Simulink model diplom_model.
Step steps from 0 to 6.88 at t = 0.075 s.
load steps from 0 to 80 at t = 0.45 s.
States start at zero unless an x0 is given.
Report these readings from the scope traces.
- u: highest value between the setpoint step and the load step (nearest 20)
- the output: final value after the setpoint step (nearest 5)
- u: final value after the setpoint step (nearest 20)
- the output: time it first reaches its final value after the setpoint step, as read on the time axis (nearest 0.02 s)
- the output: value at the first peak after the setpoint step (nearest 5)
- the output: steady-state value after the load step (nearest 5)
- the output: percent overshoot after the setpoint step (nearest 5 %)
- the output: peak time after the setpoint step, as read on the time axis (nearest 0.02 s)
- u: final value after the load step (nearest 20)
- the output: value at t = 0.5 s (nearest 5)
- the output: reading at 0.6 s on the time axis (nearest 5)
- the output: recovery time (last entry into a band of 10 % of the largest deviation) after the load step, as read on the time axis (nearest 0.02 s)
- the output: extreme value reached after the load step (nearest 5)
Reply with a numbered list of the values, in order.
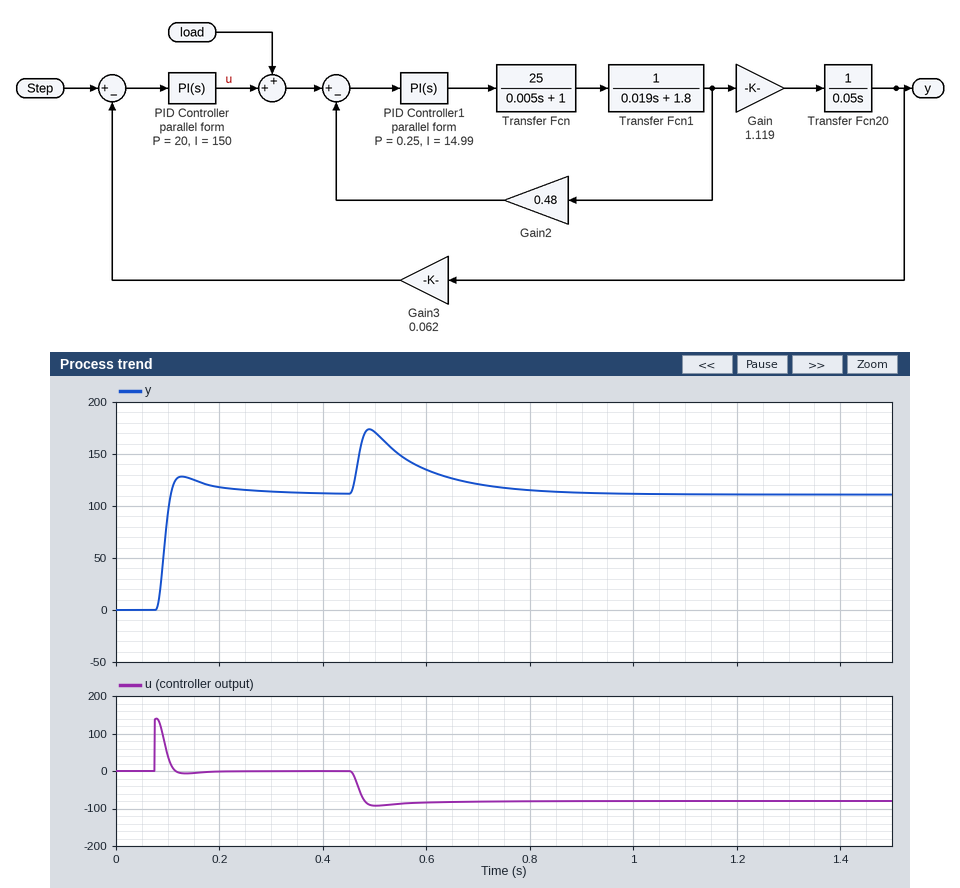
1. 140
2. 110
3. 0
4. 0.10 s
5. 130
6. 110
7. 15 %
8. 0.12 s
9. -80
10. 170
11. 135
12. 0.76 s
13. 175
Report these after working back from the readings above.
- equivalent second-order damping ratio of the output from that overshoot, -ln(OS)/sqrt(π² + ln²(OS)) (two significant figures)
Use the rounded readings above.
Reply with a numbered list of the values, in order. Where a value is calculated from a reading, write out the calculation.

1. ln(0.15) = -1.897; 1.897 / sqrt(9.870 + 3.599) = 0.52
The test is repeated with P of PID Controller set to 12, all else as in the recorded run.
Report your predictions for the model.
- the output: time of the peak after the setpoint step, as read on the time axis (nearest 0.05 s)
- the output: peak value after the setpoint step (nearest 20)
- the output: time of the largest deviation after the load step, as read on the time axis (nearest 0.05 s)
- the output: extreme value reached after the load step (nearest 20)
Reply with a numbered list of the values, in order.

1. 0.15 s
2. 140
3. 0.50 s
4. 200
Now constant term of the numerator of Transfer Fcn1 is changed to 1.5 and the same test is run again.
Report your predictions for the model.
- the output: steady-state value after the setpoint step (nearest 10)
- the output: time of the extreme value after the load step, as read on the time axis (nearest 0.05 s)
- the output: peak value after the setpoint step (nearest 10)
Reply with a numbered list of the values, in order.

1. 110
2. 0.50 s
3. 120
